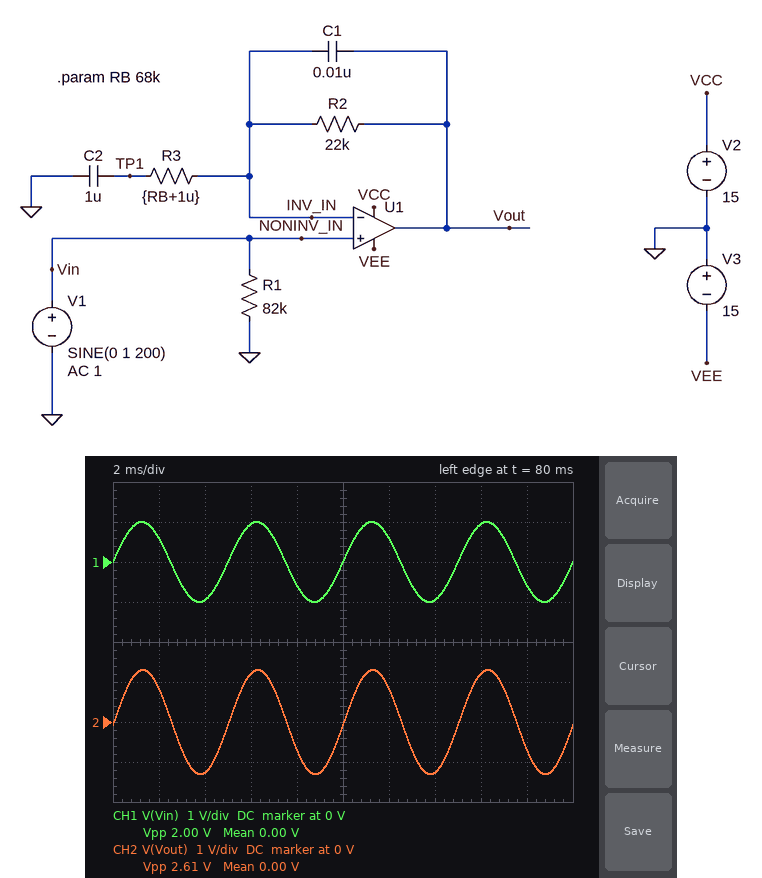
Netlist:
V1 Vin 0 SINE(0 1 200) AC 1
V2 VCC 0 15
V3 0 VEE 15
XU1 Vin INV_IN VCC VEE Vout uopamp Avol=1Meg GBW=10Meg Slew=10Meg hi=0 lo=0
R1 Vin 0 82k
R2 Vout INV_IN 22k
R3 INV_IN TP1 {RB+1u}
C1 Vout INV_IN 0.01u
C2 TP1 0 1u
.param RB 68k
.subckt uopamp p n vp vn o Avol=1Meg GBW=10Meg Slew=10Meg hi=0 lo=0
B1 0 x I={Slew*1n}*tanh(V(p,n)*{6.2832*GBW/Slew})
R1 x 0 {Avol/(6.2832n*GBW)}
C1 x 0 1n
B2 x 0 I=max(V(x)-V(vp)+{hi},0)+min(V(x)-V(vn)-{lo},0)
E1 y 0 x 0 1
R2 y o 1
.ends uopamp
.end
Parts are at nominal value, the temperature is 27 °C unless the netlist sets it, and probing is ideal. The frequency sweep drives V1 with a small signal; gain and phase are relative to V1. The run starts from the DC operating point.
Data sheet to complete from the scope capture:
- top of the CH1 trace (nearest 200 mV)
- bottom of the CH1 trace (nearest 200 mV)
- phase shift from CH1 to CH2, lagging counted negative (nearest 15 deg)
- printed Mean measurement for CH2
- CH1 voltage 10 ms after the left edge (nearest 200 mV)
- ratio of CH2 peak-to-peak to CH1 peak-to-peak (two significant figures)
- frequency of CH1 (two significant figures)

1.0 V
-1.0 V
0 deg
0.00 V
0 V
1.3
200 Hz
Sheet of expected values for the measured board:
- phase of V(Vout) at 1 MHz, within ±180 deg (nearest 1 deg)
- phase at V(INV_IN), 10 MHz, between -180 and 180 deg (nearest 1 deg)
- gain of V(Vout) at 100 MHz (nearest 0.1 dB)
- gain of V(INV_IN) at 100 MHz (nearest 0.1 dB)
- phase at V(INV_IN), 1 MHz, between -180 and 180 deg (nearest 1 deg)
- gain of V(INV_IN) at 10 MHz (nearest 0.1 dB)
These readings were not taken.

-6 deg
-45 deg
-20.0 dB
-20.0 dB
-6 deg
-3.0 dB
